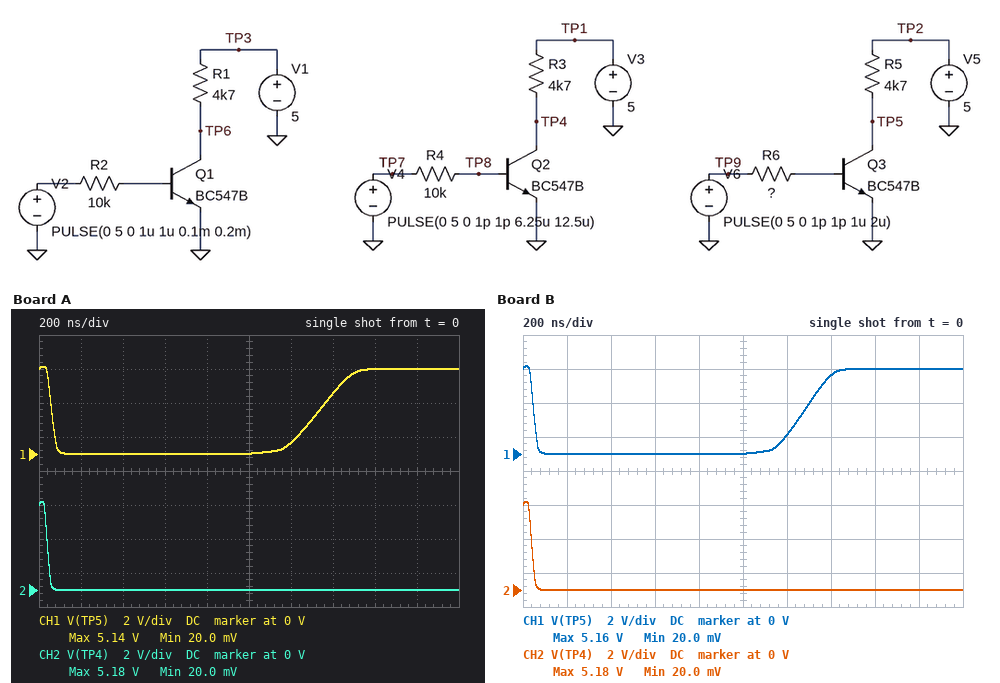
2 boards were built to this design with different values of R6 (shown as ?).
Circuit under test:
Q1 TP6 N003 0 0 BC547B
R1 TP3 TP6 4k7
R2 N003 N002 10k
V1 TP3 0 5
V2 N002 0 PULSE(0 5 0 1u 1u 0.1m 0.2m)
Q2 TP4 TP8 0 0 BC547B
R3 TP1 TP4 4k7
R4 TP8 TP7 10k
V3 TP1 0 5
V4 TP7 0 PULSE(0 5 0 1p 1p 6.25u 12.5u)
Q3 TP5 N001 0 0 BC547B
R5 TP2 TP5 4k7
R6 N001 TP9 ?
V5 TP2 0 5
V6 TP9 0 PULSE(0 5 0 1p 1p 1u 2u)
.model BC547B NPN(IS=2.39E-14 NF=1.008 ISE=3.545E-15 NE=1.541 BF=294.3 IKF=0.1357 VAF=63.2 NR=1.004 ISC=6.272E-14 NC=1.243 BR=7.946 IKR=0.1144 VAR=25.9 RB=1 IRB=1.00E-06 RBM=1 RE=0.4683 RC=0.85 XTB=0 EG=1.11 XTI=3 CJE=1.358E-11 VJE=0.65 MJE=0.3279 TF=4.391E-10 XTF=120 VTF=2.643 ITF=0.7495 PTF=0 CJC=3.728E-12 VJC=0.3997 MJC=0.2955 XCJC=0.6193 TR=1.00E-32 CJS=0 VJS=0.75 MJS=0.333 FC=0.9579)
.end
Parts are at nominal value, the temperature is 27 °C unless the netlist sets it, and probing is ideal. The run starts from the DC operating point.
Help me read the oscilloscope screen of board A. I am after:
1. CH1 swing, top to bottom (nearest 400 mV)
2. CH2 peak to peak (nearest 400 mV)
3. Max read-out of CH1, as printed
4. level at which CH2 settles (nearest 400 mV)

5.2 V
5.2 V
5.14 V
0 V
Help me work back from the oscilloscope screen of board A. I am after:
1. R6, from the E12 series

15 kΩ
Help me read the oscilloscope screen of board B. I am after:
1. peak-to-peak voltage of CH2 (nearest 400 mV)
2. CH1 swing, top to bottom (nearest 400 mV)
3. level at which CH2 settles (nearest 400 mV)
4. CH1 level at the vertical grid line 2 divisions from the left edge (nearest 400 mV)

5.2 V
5.2 V
0 V
0 V
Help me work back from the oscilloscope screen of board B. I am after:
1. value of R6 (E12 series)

12 kΩ
